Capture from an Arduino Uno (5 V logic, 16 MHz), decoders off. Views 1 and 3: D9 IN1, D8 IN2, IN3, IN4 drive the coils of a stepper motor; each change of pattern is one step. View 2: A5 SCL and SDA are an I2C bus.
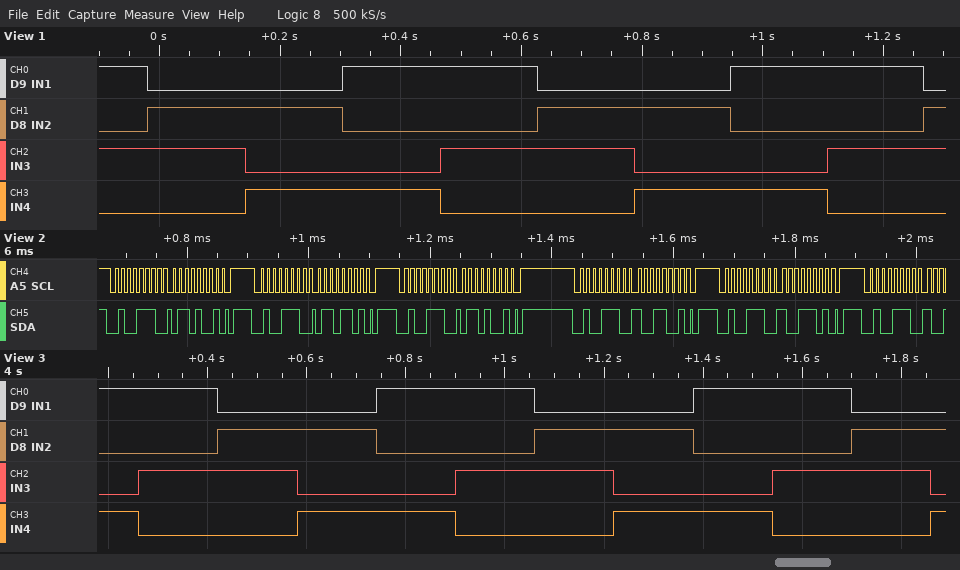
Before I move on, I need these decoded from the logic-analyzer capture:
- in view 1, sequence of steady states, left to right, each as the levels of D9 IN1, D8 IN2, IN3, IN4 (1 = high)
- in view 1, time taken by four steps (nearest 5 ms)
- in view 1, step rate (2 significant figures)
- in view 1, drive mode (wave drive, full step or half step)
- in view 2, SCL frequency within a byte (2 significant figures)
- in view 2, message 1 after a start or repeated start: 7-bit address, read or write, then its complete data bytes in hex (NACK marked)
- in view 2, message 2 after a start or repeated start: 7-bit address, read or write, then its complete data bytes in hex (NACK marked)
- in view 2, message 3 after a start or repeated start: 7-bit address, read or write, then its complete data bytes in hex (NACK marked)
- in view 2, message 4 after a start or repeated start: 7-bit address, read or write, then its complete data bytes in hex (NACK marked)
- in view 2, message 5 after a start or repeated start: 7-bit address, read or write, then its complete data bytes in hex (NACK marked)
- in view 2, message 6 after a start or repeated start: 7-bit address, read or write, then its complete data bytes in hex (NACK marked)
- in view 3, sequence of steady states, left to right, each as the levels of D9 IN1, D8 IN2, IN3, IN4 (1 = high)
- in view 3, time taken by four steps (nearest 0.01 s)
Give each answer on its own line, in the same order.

1010 0110 0101 1001 1010 0110 0101 1001 1010 0110
645 ms
6.2 steps/s
full step
100 kHz
0x27 write: 69
0x27 write: 6D
0x27 write: 69
0x27 write: 99
0x27 write: 9D
0x27 write
1001 1010 0110 0101 1001 1010 0110 0101 1001 1010 0110 0101
0.64 s
